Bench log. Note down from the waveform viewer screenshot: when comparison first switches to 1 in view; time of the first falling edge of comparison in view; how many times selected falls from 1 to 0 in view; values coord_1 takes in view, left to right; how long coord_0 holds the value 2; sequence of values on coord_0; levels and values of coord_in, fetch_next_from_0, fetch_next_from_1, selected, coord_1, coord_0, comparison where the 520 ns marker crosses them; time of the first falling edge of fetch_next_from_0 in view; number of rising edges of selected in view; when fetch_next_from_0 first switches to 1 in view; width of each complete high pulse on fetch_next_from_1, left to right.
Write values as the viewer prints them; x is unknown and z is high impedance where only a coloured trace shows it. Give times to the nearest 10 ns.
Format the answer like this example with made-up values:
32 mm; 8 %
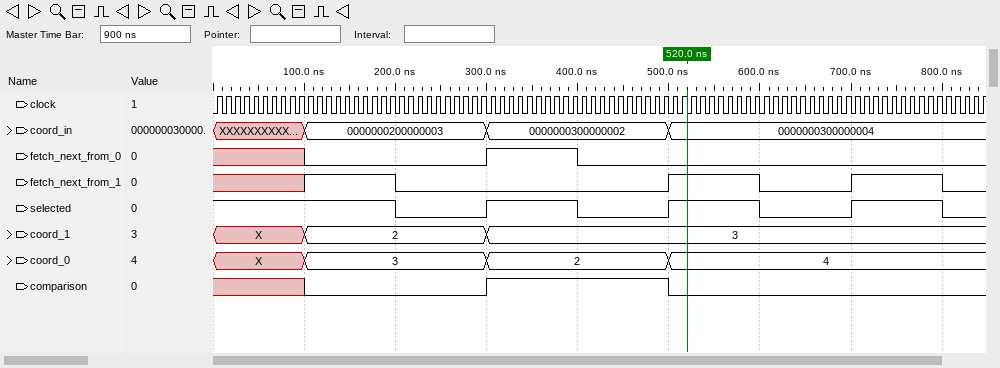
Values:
300 ns; 500 ns; 4; X, 2, 3; 200 ns; X, 3, 2, 4; coord_in=0000000300000004, fetch_next_from_0=0, fetch_next_from_1=1, selected=1, coord_1=3, coord_0=4, comparison=0; 400 ns; 3; 300 ns; 100 ns, 100 ns
